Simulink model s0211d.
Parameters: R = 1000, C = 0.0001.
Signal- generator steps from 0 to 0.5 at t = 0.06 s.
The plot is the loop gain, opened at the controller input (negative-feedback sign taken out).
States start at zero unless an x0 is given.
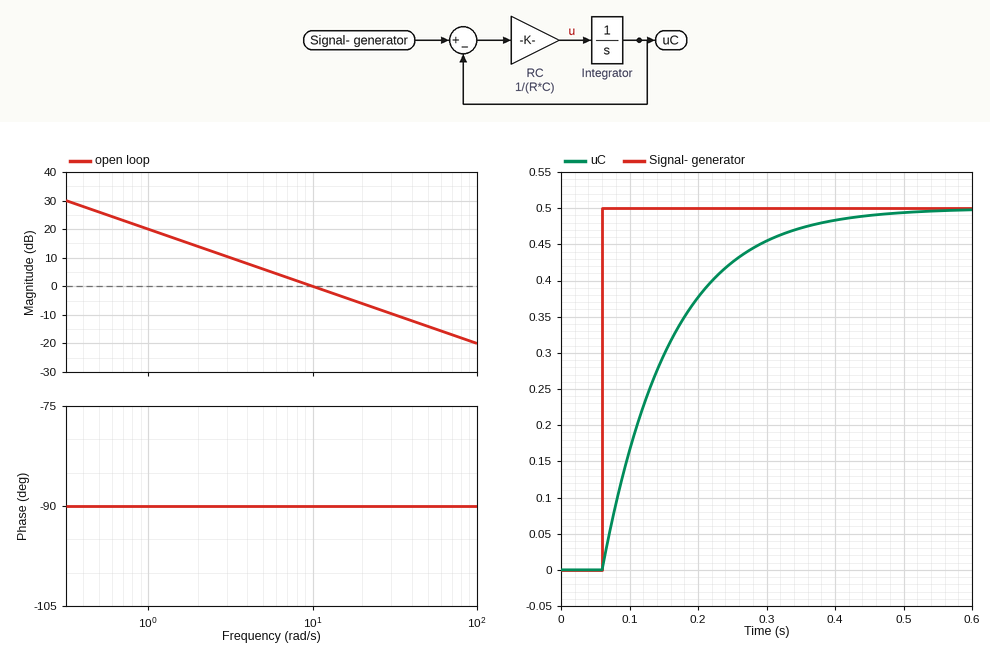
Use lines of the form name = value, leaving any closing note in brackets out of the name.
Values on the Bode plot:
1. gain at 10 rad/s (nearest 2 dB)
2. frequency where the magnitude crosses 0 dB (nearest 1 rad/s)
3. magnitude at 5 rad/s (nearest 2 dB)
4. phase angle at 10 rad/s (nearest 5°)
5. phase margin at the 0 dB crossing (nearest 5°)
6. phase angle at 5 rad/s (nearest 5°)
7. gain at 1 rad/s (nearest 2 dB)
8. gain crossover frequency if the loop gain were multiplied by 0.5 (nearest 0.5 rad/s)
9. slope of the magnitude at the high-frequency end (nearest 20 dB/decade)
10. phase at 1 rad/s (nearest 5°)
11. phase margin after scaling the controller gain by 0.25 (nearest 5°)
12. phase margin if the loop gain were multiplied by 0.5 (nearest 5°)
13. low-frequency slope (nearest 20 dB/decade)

gain at 10 rad/s = 0 dB
frequency where the magnitude crosses 0 dB = 10 rad/s
magnitude at 5 rad/s = 6 dB
phase angle at 10 rad/s = -90°
phase margin at the 0 dB crossing = 90°
phase angle at 5 rad/s = -90°
gain at 1 rad/s = 20 dB
gain crossover frequency if the loop gain were multiplied by 0.5 = 5.0 rad/s
slope of the magnitude at the high-frequency end = -20 dB/decade
phase at 1 rad/s = -90°
phase margin after scaling the controller gain by 0.25 = 90°
phase margin if the loop gain were multiplied by 0.5 = 90°
low-frequency slope = -20 dB/decade
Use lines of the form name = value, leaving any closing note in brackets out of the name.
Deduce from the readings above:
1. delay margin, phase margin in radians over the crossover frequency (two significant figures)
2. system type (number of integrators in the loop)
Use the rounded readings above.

delay margin, phase margin in radians over the crossover frequency = 0.16 s
system type = 1
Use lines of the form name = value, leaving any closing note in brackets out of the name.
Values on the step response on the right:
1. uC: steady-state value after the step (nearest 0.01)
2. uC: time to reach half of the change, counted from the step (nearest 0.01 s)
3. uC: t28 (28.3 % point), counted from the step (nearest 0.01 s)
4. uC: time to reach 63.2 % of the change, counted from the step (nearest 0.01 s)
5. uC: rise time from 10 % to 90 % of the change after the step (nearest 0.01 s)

uC: steady-state value after the step = 0.50
uC: time to reach half of the change, counted from the step = 0.07 s
uC: t28 (28.3 % point), counted from the step = 0.03 s
uC: time to reach 63.2 % of the change, counted from the step = 0.10 s
uC: rise time from 10 % to 90 % of the change after the step = 0.22 s
